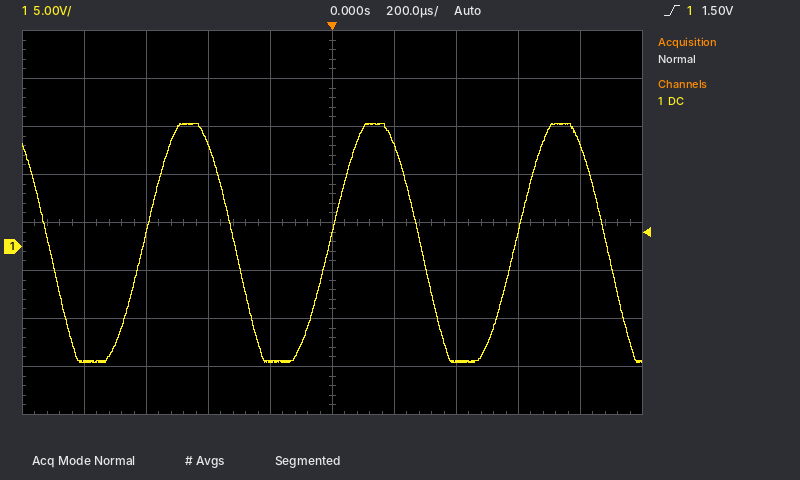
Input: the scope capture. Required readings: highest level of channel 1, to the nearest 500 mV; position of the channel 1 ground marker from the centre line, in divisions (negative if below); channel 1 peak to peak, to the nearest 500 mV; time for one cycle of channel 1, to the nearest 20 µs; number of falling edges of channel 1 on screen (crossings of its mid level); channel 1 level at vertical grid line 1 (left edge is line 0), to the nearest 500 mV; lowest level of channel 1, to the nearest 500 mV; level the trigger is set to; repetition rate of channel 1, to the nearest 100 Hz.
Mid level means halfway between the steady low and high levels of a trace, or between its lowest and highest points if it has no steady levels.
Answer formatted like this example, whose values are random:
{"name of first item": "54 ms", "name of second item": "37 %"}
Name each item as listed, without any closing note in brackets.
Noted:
{"highest level of channel 1, to the nearest 500 mV": "13.0 V", "position of the channel 1 ground marker from the centre line, in divisions": "-0.5 div", "channel 1 peak to peak, to the nearest 500 mV": "25.0 V", "time for one cycle of channel 1, to the nearest 20 µs": "600 µs", "number of falling edges of channel 1 on screen": "4", "channel 1 level at vertical grid line 1 (left edge is line 0), to the nearest 500 mV": "-12.0 V", "lowest level of channel 1, to the nearest 500 mV": "-12.0 V", "level the trigger is set to": "1.50 V", "repetition rate of channel 1, to the nearest 100 Hz": "1.7 kHz"}
